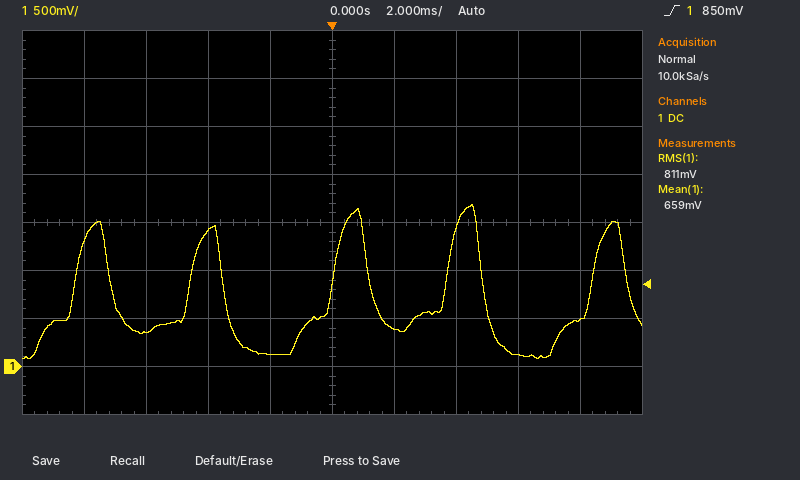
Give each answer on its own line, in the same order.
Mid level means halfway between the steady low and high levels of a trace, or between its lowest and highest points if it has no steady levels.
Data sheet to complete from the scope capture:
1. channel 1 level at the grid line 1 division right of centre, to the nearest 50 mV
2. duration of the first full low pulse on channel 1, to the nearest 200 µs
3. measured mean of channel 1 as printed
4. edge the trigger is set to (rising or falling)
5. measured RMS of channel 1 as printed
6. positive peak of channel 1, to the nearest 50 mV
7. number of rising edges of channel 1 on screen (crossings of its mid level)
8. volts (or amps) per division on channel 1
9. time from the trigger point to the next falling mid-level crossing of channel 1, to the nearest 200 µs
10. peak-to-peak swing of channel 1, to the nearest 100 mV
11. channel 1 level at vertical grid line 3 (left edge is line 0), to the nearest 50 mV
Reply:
400 mV
2.6 ms
659 mV
rising
811 mV
1.70 V
5
500 mV
1.2 ms
1.60 V
1.40 V
